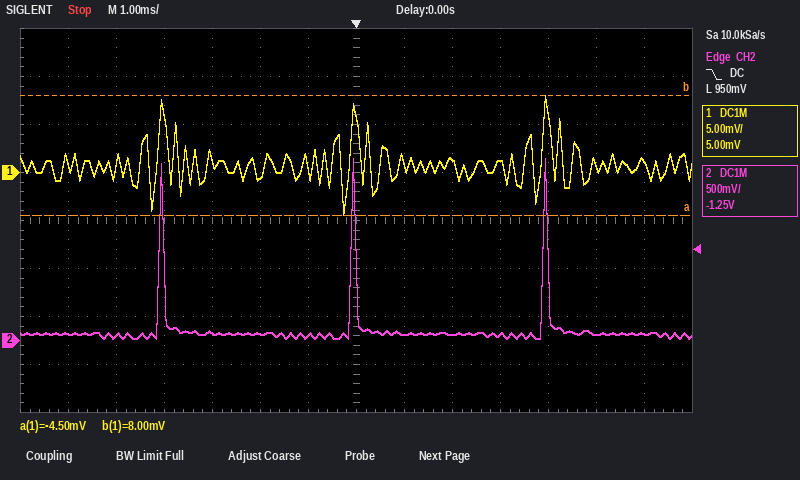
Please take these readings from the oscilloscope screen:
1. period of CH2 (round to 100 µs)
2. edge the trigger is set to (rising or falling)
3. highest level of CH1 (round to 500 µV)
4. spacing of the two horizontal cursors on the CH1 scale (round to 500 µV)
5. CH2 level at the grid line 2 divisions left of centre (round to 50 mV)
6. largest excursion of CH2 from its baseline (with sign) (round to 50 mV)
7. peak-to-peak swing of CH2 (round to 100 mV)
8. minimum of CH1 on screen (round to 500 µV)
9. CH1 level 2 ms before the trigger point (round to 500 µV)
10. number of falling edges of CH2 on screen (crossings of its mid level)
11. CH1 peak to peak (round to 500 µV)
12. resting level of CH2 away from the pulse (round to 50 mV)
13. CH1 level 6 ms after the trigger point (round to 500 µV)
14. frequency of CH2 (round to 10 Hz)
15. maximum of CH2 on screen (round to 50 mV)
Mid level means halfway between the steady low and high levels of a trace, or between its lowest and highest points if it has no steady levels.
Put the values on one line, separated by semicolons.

4.0 ms; falling; 8.0 mV; 12.5 mV; 50 mV; +1.85 V; 1.90 V; -4.5 mV; -500 µV; 3; 12.5 mV; 50 mV; 1.0 mV; 250 Hz; 1.90 V
